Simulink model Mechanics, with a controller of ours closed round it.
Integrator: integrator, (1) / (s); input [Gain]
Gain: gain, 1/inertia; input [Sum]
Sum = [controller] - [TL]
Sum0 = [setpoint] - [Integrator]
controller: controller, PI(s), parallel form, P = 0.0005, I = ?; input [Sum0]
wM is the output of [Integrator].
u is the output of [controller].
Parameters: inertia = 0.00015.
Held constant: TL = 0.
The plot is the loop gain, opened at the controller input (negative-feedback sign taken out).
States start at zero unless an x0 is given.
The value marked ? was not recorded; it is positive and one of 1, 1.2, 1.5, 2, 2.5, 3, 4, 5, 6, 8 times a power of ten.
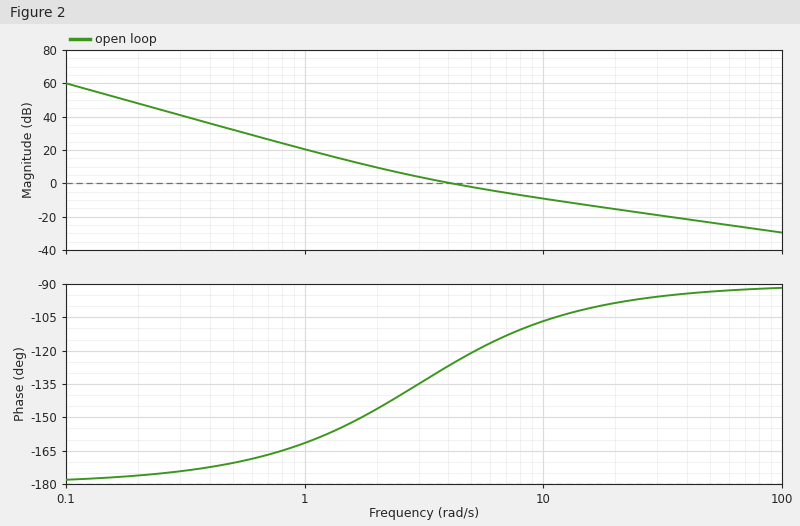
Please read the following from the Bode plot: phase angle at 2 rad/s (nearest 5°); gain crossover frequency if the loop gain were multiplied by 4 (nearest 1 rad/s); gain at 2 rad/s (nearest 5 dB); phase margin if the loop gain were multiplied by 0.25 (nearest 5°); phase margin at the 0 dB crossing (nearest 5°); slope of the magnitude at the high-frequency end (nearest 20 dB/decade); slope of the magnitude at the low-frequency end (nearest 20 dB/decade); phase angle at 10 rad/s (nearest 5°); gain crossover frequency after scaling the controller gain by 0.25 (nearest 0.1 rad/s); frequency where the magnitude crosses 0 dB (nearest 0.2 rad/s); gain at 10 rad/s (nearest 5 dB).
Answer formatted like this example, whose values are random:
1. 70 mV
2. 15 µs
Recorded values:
1. -145°
2. 14 rad/s
3. 10 dB
4. 30°
5. 55°
6. -20 dB/decade
7. -40 dB/decade
8. -105°
9. 1.7 rad/s
10. 4.2 rad/s
11. -10 dB
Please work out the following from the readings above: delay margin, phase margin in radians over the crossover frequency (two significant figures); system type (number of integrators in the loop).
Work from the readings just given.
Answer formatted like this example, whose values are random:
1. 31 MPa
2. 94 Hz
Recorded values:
1. 0.23 s
2. 2
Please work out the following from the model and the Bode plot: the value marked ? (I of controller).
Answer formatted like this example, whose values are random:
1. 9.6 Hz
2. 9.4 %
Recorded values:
1. 0.0015
